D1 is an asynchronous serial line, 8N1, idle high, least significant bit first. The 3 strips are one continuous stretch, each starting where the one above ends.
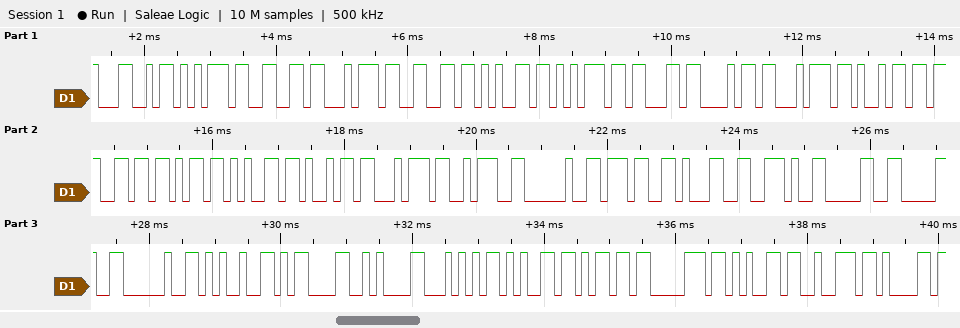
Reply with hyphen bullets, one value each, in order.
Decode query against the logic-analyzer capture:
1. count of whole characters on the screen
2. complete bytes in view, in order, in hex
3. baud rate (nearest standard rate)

- 34
- 4C 75 66 74 66 65 75 63 68 74 69 67 6B 65 69 74 3A 20 37 31 2E 30 30 20 25 0D 0A 54 65 6D 70 65 72 61
- 9600 baud
